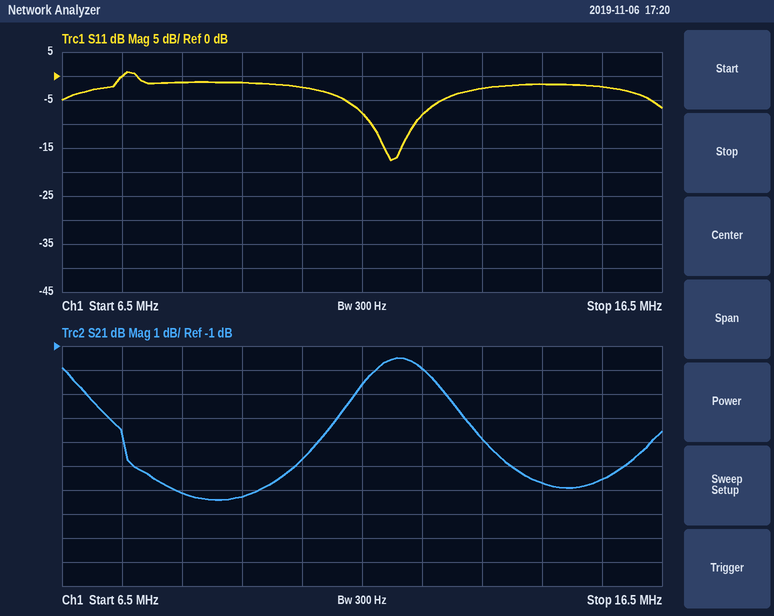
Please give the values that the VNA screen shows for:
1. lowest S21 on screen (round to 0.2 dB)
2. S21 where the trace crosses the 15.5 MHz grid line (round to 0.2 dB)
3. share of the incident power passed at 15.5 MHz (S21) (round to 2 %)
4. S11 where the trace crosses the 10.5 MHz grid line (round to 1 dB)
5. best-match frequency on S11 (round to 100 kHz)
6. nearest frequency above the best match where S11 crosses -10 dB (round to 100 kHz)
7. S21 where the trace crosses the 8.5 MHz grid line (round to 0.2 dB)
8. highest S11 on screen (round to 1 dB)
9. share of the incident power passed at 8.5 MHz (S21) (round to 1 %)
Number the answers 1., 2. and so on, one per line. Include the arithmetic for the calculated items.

1. -7.4 dB
2. -6.6 dB
3. 10^(-6.6/10) ≈ 22 %
4. -2 dB
5. 12.0 MHz
6. 12.4 MHz
7. -7.2 dB
8. 1 dB
9. 10^(-7.2/10) ≈ 19 %
